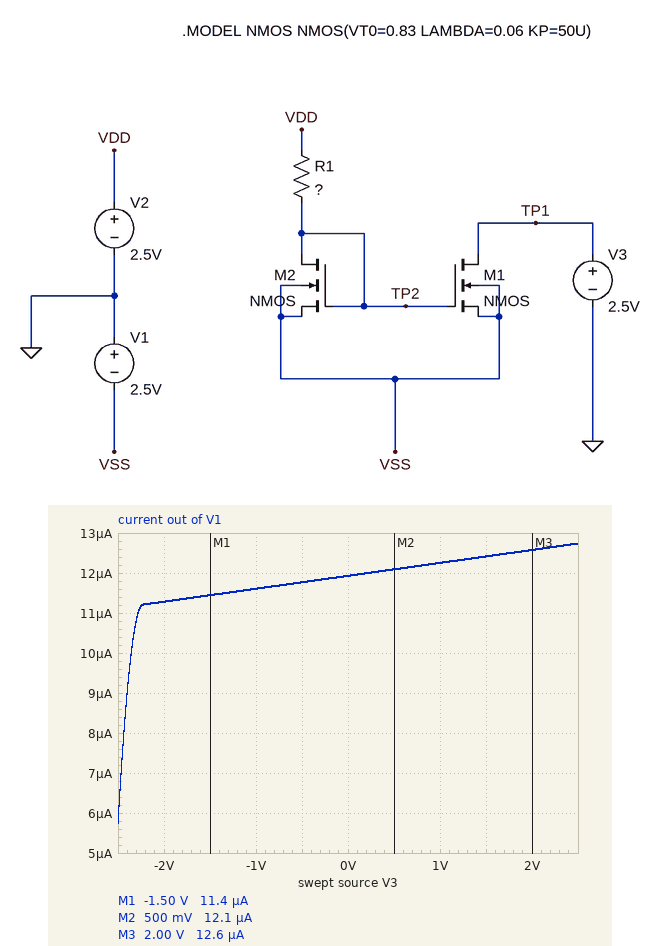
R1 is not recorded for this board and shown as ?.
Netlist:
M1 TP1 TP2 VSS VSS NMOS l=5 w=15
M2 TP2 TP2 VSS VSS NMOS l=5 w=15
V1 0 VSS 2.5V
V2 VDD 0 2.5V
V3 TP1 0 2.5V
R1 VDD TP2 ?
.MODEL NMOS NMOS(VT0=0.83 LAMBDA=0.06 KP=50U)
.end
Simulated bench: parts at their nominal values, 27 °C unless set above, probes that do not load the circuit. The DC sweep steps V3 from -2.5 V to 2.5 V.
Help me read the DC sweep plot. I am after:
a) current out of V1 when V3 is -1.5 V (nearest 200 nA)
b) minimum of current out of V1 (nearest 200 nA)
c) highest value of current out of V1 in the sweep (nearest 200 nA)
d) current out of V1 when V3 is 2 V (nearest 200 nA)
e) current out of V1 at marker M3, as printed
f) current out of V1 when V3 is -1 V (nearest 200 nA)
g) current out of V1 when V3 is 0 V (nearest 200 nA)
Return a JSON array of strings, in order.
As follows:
["11.4 µA", "5.8 µA", "12.8 µA", "12.6 µA", "12.6 µA", "11.6 µA", "12.0 µA"]
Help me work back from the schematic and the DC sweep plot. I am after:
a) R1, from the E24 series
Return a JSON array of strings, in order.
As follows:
["680 kΩ"]
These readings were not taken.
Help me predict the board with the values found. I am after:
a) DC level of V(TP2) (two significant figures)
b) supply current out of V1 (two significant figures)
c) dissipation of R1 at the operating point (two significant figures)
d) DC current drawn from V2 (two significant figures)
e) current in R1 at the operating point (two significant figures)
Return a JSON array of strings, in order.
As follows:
["-1.4 V", "13 µA", "22 µW", "5.7 µA", "5.7 µA"]
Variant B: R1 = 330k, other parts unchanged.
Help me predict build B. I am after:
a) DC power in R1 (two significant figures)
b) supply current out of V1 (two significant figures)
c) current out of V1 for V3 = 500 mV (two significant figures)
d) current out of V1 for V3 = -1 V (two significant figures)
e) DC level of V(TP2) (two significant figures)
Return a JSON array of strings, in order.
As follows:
["44 µW", "25 µA", "24 µA", "23 µA", "-1.3 V"]
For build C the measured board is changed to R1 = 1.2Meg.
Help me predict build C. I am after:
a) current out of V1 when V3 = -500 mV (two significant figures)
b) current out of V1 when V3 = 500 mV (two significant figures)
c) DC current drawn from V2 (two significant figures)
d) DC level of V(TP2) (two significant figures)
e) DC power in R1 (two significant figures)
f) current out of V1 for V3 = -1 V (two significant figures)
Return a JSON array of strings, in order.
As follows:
["6.8 µA", "7.0 µA", "3.3 µA", "-1.5 V", "13 µW", "6.7 µA"]
